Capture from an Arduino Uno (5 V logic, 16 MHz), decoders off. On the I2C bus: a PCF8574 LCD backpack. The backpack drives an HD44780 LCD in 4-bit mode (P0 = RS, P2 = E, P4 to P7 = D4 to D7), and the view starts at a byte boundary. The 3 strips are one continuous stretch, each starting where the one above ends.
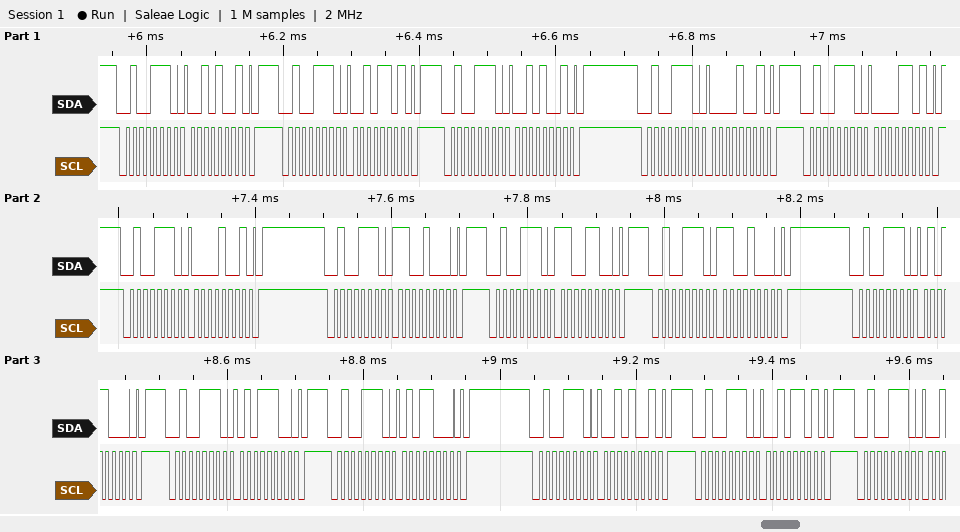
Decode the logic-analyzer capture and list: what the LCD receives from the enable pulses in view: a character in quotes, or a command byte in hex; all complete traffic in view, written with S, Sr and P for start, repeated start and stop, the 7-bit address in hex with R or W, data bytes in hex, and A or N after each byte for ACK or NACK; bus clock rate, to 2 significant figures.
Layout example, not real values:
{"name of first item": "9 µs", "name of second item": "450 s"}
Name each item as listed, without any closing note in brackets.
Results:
{"what the LCD receives from the enable pulses in view: a character in quotes, or a command byte in hex": "' ' 0xC5", "all complete traffic in view, written with S, Sr and P for start, repeated start and stop, the 7-bit address in hex with R or W, data bytes in hex, and A or N after each byte for ACK or NACK": "S 27W A 29 A P S 27W A 2D A P S 27W A 29 A P S 27W A 09 A P S 27W A 0D A P S 27W A 09 A P S 27W A C8 A P S 27W A CC A P S 27W A C8 A P S 27W A 58 A P S 27W A 5C A P S 27W A 58 A P S 27W A 29 A P S 27W A 2D A P S 27W A", "bus clock rate, to 2 significant figures": "100 kHz"}
